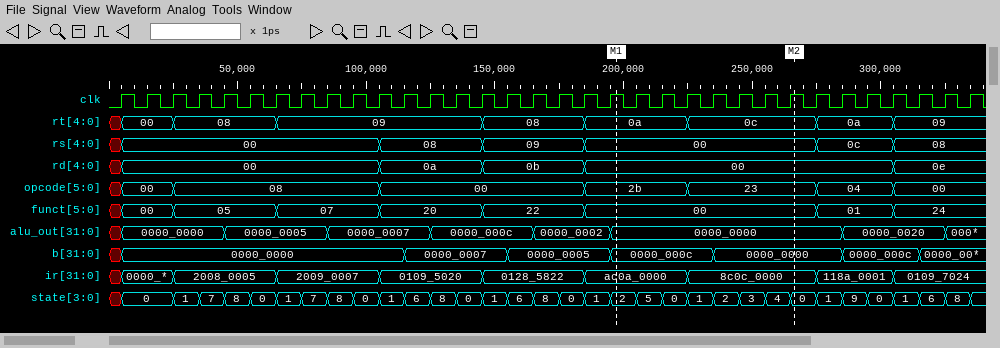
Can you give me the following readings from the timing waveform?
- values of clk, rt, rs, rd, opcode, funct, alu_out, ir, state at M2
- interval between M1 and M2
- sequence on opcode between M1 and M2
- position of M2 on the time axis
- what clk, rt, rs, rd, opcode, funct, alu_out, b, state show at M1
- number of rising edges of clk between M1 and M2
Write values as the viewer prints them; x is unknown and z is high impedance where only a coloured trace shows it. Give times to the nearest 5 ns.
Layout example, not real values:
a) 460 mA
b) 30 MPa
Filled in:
a) clk=1, rt=0c, rs=00, rd=00, opcode=23, funct=00, alu_out=0000_0000, ir=8c0c_0000, state=0
b) 70 ns
c) 2b, 23
d) 265 ns
e) clk=1, rt=0a, rs=00, rd=00, opcode=2b, funct=00, alu_out=0000_0000, b=0000_000c, state=2
f) 7
